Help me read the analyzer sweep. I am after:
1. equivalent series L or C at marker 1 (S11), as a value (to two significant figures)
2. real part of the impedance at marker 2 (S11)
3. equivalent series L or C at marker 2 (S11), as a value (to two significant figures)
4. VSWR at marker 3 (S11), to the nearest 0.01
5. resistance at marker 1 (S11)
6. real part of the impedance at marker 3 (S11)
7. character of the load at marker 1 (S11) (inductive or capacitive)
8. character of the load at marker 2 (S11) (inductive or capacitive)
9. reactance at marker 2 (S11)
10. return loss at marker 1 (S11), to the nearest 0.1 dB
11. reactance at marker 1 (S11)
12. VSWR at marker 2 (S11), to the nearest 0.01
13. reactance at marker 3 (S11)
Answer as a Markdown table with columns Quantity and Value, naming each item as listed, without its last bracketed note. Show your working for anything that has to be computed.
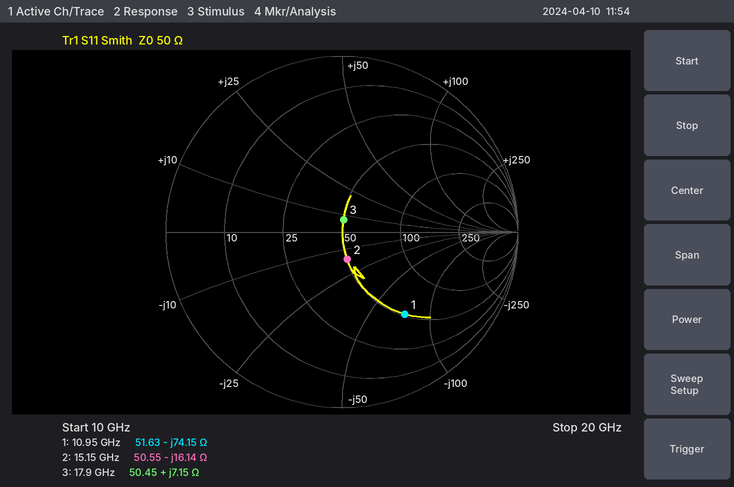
| Quantity | Value |
|---|---|
| equivalent series L or C at marker 1 (S11), as a value | C = 1/(2π × 10.95 GHz × 74.15 Ω) ≈ 196 fF, so 200 fF to two significant figures |
| real part of the impedance at marker 2 | 50.55 Ω |
| equivalent series L or C at marker 2 (S11), as a value | C = 1/(2π × 15.15 GHz × 16.14 Ω) ≈ 651 fF, so 650 fF to two significant figures |
| VSWR at marker 3 (S11), to the nearest 0.01 | 1.15 |
| resistance at marker 1 | 51.63 Ω |
| real part of the impedance at marker 3 | 50.45 Ω |
| character of the load at marker 1 (S11) | capacitive |
| character of the load at marker 2 (S11) | capacitive |
| reactance at marker 2 | -16.14 Ω |
| return loss at marker 1 (S11), to the nearest 0.1 dB | 4.6 dB |
| reactance at marker 1 | -74.15 Ω |
| VSWR at marker 2 (S11), to the nearest 0.01 | 1.38 |
| reactance at marker 3 | +7.15 Ω |
